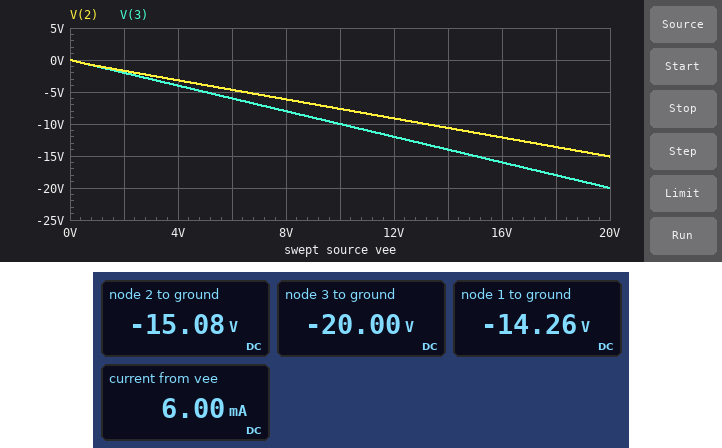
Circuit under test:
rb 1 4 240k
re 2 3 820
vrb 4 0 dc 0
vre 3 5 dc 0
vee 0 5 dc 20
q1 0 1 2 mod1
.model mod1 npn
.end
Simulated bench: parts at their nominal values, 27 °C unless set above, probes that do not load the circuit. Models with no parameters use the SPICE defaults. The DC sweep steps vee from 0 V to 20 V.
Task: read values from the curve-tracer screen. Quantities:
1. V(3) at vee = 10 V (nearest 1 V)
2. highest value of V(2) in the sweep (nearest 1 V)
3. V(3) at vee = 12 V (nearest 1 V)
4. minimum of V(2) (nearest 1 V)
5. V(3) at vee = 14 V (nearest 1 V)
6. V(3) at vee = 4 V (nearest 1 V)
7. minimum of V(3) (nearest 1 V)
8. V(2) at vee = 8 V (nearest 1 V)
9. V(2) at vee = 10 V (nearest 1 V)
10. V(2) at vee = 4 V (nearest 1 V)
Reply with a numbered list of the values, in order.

1. -10 V
2. 0 V
3. -12 V
4. -15 V
5. -14 V
6. -4 V
7. -20 V
8. -6 V
9. -8 V
10. -3 V
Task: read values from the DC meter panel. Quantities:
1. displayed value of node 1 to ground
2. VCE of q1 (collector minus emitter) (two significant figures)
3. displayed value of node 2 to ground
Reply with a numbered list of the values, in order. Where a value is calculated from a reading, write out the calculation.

1. -14.26 V
2. 0 V - (-15.08 V) = 15 V
3. -15.08 V
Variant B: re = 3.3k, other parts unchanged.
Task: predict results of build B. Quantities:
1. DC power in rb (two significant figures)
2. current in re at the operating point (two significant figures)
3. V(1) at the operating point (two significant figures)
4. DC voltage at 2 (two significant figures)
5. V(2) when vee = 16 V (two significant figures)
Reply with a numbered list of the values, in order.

1. 270 µW
2. 3.4 mA
3. -8.0 V
4. -8.8 V
5. -7.2 V
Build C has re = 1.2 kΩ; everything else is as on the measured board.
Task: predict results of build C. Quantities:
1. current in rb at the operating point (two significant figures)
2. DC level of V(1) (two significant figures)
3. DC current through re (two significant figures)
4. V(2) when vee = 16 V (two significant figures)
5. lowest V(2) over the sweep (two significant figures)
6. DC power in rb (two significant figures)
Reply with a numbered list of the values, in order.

1. 53 µA
2. -13 V
3. 5.4 mA
4. -11 V
5. -14 V
6. 680 µW
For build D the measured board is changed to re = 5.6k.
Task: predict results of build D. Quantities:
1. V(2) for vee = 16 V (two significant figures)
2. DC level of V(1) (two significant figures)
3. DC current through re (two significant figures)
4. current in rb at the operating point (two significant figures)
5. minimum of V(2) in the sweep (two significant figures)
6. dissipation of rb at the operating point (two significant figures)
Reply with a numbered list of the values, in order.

1. -5.3 V
2. -5.7 V
3. 2.4 mA
4. 24 µA
5. -6.5 V
6. 140 µW
